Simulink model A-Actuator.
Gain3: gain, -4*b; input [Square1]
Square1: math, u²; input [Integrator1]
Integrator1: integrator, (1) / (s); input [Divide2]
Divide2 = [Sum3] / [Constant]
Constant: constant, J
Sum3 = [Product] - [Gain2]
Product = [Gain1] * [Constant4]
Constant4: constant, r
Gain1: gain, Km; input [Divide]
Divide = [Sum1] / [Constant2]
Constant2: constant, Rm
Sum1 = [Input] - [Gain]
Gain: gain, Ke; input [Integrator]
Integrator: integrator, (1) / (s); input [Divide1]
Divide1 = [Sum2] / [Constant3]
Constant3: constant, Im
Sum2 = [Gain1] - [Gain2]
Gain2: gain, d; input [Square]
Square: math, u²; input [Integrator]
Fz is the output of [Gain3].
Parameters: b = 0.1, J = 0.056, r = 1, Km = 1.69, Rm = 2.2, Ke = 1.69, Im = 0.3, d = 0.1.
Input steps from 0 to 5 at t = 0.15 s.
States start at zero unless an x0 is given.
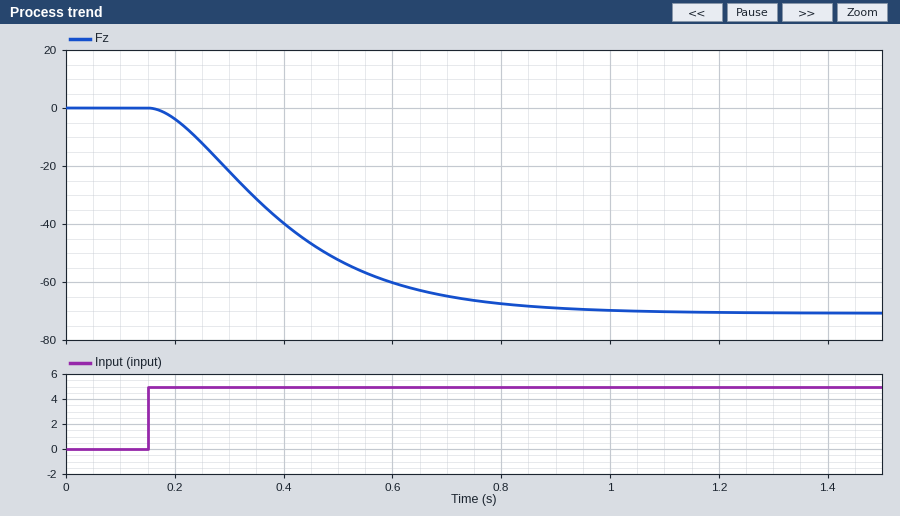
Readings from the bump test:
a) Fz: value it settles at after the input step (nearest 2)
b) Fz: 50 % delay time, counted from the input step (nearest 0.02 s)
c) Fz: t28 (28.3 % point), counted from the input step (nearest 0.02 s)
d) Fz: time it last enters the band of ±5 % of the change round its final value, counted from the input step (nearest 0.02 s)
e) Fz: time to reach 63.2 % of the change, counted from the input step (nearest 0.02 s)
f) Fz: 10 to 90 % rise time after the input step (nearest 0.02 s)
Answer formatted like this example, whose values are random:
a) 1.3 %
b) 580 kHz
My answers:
a) -70
b) 0.22 s
c) 0.14 s
d) 0.64 s
e) 0.28 s
f) 0.44 s
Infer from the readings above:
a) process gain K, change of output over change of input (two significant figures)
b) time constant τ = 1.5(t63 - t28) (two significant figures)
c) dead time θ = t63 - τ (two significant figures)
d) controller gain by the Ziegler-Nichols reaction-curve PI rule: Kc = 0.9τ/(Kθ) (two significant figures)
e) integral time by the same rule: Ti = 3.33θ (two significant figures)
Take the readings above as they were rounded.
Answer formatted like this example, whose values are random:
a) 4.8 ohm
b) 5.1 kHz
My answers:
a) -14
b) 0.21 s
c) 0.070 s
d) -0.19
e) 0.23 s
